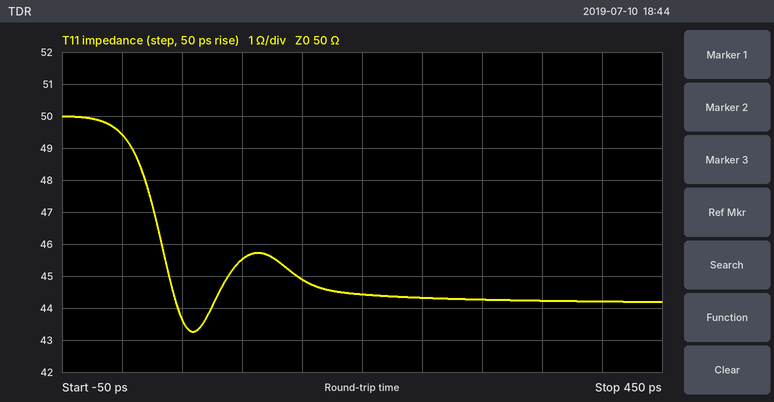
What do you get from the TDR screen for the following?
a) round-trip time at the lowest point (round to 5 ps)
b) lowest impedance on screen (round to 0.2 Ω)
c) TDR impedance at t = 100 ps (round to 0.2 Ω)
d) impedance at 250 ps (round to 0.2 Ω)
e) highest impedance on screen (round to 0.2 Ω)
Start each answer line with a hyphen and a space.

- 60 ps
- 43.2 Ω
- 45.6 Ω
- 44.4 Ω
- 50.0 Ω
